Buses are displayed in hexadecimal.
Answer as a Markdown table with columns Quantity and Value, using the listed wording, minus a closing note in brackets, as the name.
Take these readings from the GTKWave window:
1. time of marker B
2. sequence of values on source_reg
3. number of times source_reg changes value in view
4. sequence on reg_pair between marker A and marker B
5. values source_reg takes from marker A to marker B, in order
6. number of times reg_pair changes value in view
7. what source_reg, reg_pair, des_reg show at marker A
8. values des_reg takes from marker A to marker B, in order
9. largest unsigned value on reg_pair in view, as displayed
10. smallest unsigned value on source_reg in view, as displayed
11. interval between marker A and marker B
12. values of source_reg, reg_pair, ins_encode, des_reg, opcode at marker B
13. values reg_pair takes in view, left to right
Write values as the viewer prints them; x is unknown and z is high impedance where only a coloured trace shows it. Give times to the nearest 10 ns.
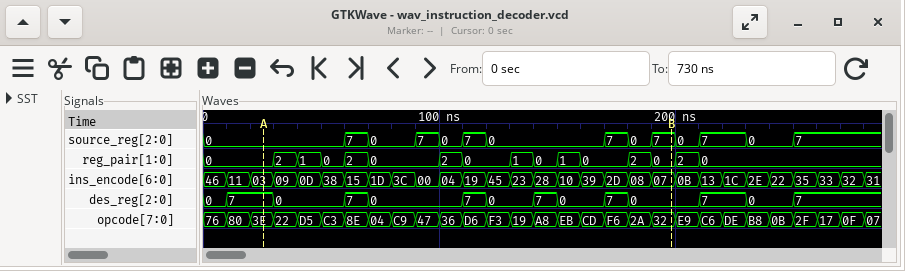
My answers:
| Quantity | Value |
|---|---|
| time of marker B | 200 ns |
| sequence of values on source_reg | 0, 7, 0, 7, 0, 7, 0, 7, 0, 7, 0, 7, 0, 7 |
| number of times source_reg changes value in view | 13 |
| sequence on reg_pair between marker A and marker B | 0, 2, 1, 0, 2, 0, 2, 0, 1, 0, 1, 0, 2, 0 |
| values source_reg takes from marker A to marker B, in order | 0, 7, 0, 7, 0, 7, 0, 7, 0, 7 |
| number of times reg_pair changes value in view | 15 |
| what source_reg, reg_pair, des_reg show at marker A | source_reg=0, reg_pair=0, des_reg=7 |
| values des_reg takes from marker A to marker B, in order | 7, 0, 7, 0, 7, 0, 7, 0, 7, 0 |
| largest unsigned value on reg_pair in view, as displayed | 2 |
| smallest unsigned value on source_reg in view, as displayed | 0 |
| interval between marker A and marker B | 170 ns |
| values of source_reg, reg_pair, ins_encode, des_reg, opcode at marker B | source_reg=7, reg_pair=0, ins_encode=07, des_reg=0, opcode=32 |
| values reg_pair takes in view, left to right | 0, 2, 1, 0, 2, 0, 2, 0, 1, 0, 1, 0, 2, 0, 2, 0 |
